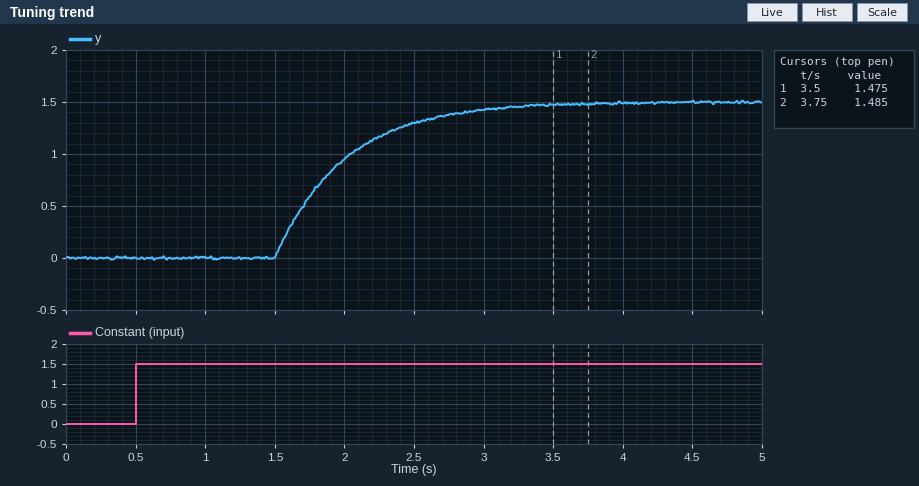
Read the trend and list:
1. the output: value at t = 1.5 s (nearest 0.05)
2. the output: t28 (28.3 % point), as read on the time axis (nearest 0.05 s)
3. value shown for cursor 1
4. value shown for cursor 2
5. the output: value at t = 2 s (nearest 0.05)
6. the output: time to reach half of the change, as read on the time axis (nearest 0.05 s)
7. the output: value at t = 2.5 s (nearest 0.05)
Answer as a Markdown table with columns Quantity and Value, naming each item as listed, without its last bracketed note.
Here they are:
| Quantity | Value |
|---|---|
| the output: value at t = 1.5 s | 0.00 |
| the output: t28 (28.3 % point), as read on the time axis | 1.65 s |
| value shown for cursor 1 | 1.475 |
| value shown for cursor 2 | 1.485 |
| the output: value at t = 2 s | 0.95 |
| the output: time to reach half of the change, as read on the time axis | 1.85 s |
| the output: value at t = 2.5 s | 1.30 |
